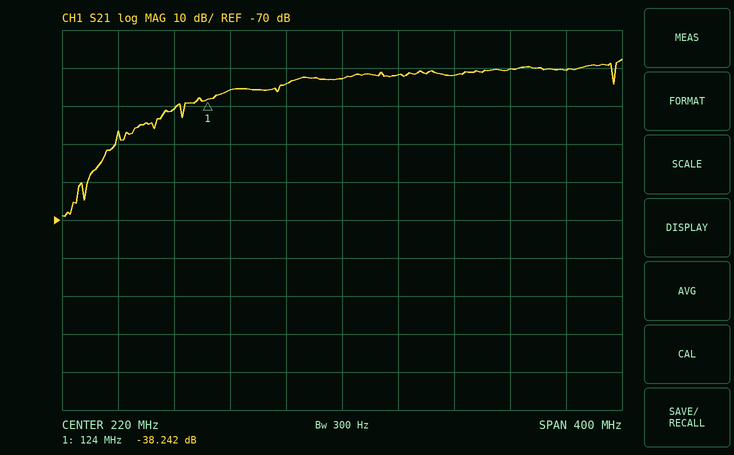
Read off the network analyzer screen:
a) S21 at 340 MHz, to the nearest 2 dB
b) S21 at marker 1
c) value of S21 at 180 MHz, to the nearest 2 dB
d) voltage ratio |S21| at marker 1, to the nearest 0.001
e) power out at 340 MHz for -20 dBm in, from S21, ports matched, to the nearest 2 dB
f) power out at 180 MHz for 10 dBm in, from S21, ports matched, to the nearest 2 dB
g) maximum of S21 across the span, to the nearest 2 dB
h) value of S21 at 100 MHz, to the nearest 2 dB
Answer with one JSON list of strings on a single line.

["-30 dB", "-38.242 dB", "-34 dB", "0.012", "-50 dBm", "-24 dBm", "-28 dB", "-40 dB"]
